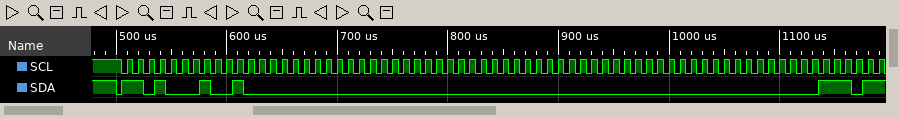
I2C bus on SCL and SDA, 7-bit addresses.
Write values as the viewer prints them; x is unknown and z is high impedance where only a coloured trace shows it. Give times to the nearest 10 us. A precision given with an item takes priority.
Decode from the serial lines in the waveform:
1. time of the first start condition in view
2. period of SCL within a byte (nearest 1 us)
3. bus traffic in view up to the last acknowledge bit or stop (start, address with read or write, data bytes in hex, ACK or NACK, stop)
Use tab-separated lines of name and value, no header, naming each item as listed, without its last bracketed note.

time of the first start condition in view	500 us
period of SCL within a byte	10 us
bus traffic in view up to the last acknowledge bit or stop	start, address 68 read ACK, 40 ACK, 00 ACK, 00 ACK, 00 ACK, 00 ACK, 00 ACK
